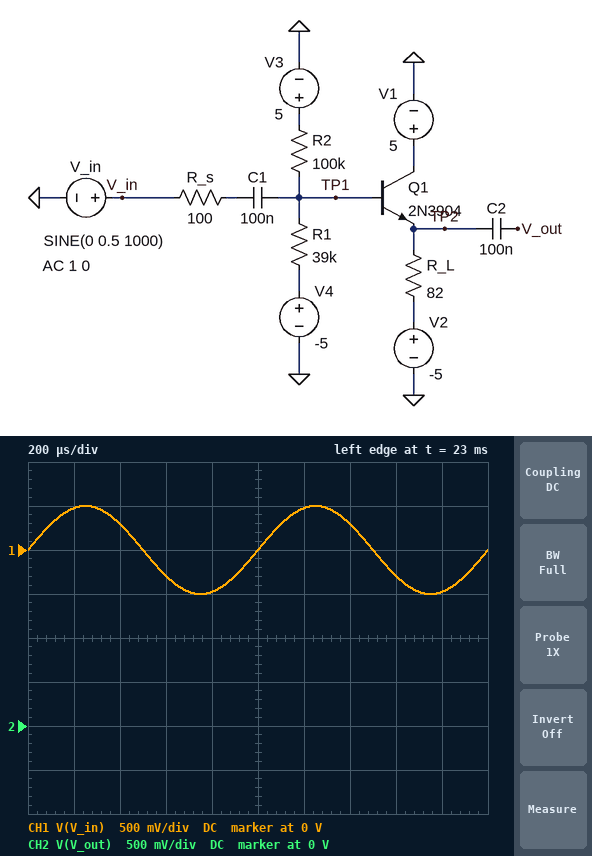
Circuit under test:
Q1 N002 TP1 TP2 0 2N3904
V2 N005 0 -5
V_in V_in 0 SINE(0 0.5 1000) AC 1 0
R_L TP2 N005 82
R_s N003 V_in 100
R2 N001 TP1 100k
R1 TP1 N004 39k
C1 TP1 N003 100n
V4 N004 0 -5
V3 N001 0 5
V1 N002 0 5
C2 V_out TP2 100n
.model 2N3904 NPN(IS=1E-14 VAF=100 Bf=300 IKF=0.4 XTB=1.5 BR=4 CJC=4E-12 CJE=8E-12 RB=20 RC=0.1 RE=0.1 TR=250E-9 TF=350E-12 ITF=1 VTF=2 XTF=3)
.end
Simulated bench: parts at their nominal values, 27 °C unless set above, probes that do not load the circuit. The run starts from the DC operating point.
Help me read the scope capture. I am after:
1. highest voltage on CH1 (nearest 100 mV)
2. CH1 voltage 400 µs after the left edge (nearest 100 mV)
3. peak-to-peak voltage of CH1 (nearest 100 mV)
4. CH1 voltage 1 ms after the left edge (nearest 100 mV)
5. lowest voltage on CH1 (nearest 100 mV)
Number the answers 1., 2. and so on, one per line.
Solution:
1. 500 mV
2. 300 mV
3. 1.0 V
4. 0 V
5. -500 mV
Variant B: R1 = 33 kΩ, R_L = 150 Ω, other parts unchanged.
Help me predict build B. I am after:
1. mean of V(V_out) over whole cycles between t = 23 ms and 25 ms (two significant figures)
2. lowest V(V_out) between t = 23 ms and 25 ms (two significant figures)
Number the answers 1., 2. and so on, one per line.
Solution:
1. -3.8 V
2. -4.3 V
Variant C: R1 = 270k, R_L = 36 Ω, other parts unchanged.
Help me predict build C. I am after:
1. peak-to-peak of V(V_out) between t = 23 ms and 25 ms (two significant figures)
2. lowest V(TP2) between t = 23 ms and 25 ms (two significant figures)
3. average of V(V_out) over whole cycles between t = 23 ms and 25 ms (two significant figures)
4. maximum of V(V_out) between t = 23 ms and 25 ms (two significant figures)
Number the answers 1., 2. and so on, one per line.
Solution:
1. 940 mV
2. -4.6 V
3. -4.1 V
4. -3.7 V
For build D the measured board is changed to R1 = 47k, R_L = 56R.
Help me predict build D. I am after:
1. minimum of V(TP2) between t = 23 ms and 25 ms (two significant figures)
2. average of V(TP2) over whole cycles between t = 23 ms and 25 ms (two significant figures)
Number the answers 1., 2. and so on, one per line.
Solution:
1. -4.6 V
2. -4.1 V
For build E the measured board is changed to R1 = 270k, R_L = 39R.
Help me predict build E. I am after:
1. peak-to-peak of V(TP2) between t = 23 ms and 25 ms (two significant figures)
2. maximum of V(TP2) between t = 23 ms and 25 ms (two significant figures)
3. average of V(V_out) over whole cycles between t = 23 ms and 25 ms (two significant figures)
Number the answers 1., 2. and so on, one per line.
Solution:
1. 940 mV
2. -3.6 V
3. -4.1 V
